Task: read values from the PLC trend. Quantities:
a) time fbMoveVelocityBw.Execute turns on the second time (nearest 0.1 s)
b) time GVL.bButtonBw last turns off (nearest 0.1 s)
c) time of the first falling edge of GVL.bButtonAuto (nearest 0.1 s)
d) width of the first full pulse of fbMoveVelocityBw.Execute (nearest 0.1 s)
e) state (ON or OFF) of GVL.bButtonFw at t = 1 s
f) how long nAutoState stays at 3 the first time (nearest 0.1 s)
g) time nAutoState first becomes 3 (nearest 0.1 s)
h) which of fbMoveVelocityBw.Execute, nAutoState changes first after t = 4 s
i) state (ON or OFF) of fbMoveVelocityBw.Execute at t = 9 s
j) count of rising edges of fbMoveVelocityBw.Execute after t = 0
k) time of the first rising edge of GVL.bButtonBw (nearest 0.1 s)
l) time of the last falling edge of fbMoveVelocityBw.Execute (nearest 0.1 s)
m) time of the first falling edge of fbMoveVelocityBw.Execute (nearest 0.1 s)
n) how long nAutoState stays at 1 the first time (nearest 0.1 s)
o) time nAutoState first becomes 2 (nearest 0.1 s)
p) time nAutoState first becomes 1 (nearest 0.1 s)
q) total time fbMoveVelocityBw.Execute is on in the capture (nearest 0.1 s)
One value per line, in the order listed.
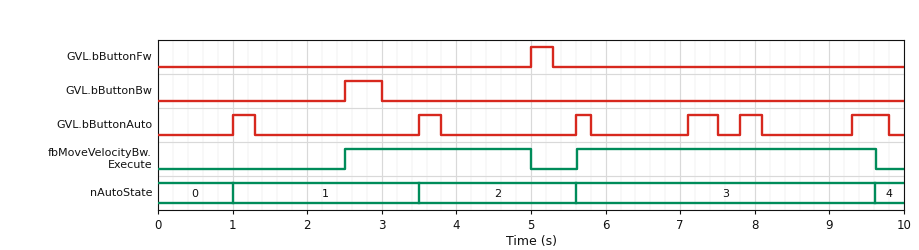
5.6 s
3.0 s
1.3 s
2.5 s
OFF
4.0 s
5.6 s
fbMoveVelocityBw.Execute
ON
2
2.5 s
9.6 s
5.0 s
2.5 s
3.5 s
1.0 s
6.5 s
